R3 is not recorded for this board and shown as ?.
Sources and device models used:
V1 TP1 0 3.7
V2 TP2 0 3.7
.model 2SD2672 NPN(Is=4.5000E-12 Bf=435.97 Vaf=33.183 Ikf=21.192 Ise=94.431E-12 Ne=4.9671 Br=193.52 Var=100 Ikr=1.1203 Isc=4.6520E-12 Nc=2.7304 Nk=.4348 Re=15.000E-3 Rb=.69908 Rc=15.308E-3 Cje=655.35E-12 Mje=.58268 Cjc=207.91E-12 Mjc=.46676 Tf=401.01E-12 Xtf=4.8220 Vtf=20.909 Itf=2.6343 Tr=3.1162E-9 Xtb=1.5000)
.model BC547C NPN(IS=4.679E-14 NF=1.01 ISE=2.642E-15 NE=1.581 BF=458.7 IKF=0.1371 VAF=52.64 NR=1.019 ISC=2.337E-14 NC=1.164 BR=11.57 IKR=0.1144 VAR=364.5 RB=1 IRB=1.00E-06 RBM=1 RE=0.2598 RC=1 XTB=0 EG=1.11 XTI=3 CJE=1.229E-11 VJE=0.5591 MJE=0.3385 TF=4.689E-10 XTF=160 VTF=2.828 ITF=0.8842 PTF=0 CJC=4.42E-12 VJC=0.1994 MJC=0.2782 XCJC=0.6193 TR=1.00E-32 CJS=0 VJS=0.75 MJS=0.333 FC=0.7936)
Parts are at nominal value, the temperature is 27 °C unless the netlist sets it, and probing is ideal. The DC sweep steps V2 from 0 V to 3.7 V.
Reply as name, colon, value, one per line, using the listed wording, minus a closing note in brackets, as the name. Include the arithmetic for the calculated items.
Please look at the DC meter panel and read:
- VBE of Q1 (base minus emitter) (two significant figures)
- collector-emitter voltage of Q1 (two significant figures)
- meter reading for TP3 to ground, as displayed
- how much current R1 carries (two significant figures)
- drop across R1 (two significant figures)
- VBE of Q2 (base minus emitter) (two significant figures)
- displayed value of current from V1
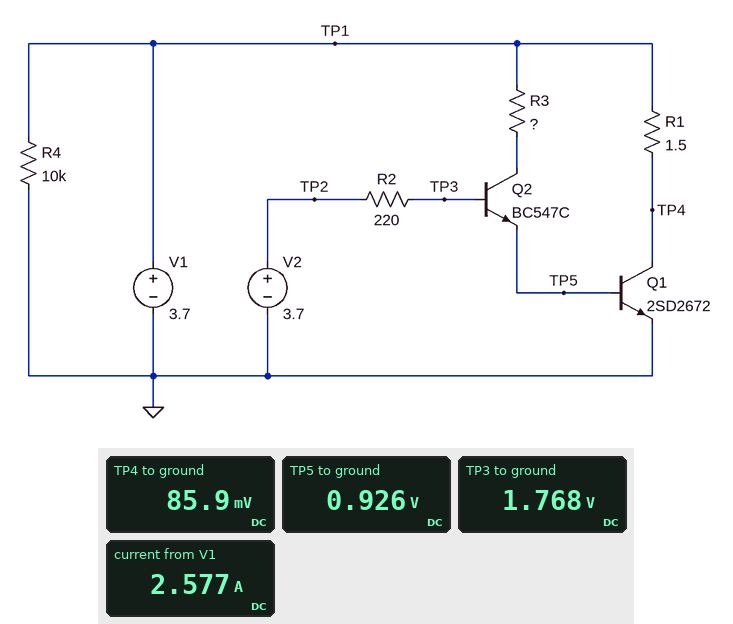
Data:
VBE of Q1 (base minus emitter): 926 mV = 930 mV
collector-emitter voltage of Q1: 85.9 mV = 86 mV
meter reading for TP3 to ground, as displayed: 1.768 V
how much current R1 carries: (3.7 V - 85.9 mV) / 1.5 Ω = 2.4 A
drop across R1: 3.7 V - 85.9 mV = 3.6 V
VBE of Q2 (base minus emitter): 1.768 V - 926 mV = 840 mV
displayed value of current from V1: 2.577 A
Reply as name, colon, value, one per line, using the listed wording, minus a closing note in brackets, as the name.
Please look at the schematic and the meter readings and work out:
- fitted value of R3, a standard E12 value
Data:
fitted value of R3, a standard E12 value: 15 Ω
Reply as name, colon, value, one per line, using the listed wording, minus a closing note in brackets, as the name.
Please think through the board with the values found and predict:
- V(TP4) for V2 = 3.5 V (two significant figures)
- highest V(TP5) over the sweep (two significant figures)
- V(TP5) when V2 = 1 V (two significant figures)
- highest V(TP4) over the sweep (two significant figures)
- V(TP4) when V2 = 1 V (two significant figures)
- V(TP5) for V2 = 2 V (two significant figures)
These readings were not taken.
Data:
V(TP4) for V2 = 3.5 V: 86 mV
highest V(TP5) over the sweep: 930 mV
V(TP5) when V2 = 1 V: 520 mV
highest V(TP4) over the sweep: 3.7 V
V(TP4) when V2 = 1 V: 3.7 V
V(TP5) for V2 = 2 V: 920 mV
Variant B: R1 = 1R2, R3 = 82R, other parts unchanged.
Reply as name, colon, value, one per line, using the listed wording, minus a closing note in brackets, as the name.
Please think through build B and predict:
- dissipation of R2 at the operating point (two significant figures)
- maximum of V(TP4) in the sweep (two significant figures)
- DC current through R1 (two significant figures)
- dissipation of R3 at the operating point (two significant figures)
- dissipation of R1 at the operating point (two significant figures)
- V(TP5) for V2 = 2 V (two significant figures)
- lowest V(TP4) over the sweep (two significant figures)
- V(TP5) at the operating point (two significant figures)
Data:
dissipation of R2 at the operating point: 20 mW
maximum of V(TP4) in the sweep: 3.7 V
DC current through R1: 3.0 A
dissipation of R3 at the operating point: 98 mW
dissipation of R1 at the operating point: 11 W
V(TP5) for V2 = 2 V: 800 mV
lowest V(TP4) over the sweep: 120 mV
V(TP5) at the operating point: 810 mV
